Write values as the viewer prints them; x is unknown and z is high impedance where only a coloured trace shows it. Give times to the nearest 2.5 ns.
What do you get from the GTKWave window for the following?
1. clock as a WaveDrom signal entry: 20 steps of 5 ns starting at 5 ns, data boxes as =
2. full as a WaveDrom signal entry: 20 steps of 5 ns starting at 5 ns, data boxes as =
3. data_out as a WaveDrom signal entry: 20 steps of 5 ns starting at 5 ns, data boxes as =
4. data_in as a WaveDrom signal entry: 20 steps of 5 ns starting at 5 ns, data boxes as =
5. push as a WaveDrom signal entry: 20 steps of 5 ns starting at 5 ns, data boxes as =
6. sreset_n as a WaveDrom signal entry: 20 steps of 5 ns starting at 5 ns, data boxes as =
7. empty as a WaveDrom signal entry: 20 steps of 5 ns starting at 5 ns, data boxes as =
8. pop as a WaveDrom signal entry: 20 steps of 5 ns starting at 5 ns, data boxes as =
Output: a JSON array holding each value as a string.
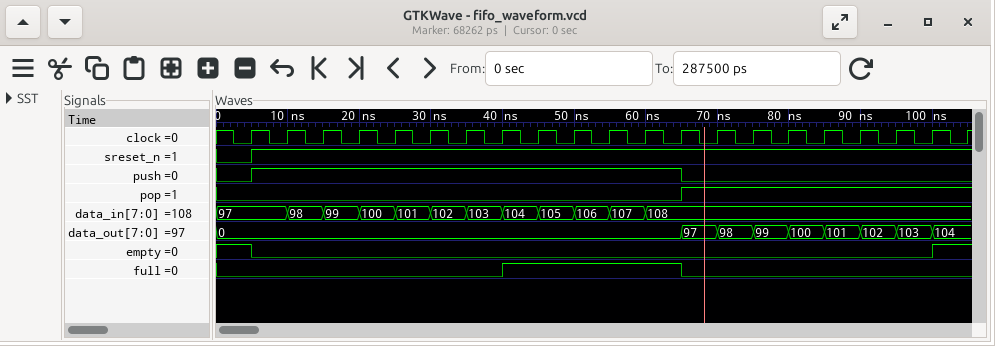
["{name: 'clock', wave: 'p...................'}", "{name: 'full', wave: '0......1....0.......'}", "{name: 'data_out', wave: '=...........========', data: '0 97 98 99 100 101 102 103 104'}", "{name: 'data_in', wave: '============........', data: '97 98 99 100 101 102 103 104 105 106 107 108'}", "{name: 'push', wave: '1...........0.......'}", "{name: 'sreset_n', wave: '1...................'}", "{name: 'empty', wave: '0..................1'}", "{name: 'pop', wave: '0...........1.......'}"]
